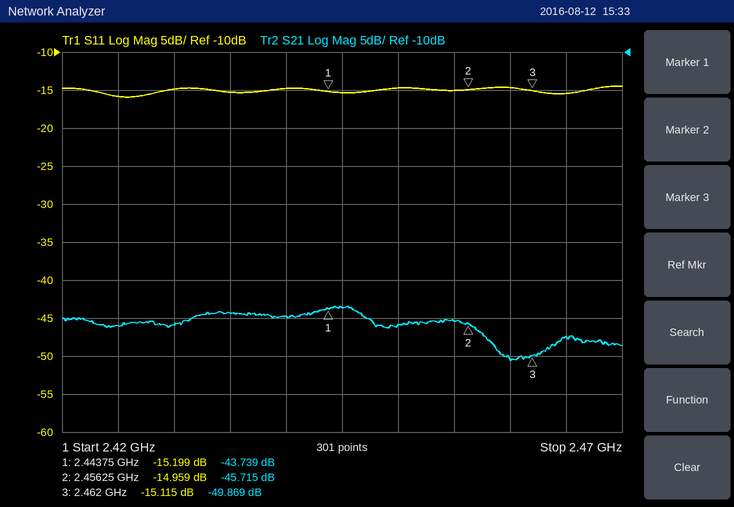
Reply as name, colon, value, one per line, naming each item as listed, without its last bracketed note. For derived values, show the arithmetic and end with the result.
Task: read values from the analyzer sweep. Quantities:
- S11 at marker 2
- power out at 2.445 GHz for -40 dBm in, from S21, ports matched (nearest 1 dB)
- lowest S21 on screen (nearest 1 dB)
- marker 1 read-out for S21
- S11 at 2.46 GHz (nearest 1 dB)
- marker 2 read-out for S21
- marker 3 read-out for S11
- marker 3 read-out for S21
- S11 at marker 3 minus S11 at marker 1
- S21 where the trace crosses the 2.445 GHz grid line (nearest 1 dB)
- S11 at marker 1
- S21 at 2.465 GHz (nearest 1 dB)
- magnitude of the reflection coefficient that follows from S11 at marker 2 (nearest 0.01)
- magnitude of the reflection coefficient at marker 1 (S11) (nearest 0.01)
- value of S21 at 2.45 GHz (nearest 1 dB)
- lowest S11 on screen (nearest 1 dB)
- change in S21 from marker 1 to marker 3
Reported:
S11 at marker 2: -14.959 dB
power out at 2.445 GHz for -40 dBm in, from S21, ports matched: -40 dBm + (-44 dB) = -84 dBm
lowest S21 on screen: -51 dB
marker 1 read-out for S21: -43.739 dB
S11 at 2.46 GHz: -15 dB
marker 2 read-out for S21: -45.715 dB
marker 3 read-out for S11: -15.115 dB
marker 3 read-out for S21: -49.869 dB
S11 at marker 3 minus S11 at marker 1: -15.115 − (-15.199) = 0.084 dB
S21 where the trace crosses the 2.445 GHz grid line: -44 dB
S11 at marker 1: -15.199 dB
S21 at 2.465 GHz: -47 dB
magnitude of the reflection coefficient that follows from S11 at marker 2: 10^(-14.959/20) ≈ 0.18
magnitude of the reflection coefficient at marker 1 (S11): 10^(-15.199/20) ≈ 0.17
value of S21 at 2.45 GHz: -46 dB
lowest S11 on screen: -16 dB
change in S21 from marker 1 to marker 3: -49.869 − (-43.739) = -6.130 dB
